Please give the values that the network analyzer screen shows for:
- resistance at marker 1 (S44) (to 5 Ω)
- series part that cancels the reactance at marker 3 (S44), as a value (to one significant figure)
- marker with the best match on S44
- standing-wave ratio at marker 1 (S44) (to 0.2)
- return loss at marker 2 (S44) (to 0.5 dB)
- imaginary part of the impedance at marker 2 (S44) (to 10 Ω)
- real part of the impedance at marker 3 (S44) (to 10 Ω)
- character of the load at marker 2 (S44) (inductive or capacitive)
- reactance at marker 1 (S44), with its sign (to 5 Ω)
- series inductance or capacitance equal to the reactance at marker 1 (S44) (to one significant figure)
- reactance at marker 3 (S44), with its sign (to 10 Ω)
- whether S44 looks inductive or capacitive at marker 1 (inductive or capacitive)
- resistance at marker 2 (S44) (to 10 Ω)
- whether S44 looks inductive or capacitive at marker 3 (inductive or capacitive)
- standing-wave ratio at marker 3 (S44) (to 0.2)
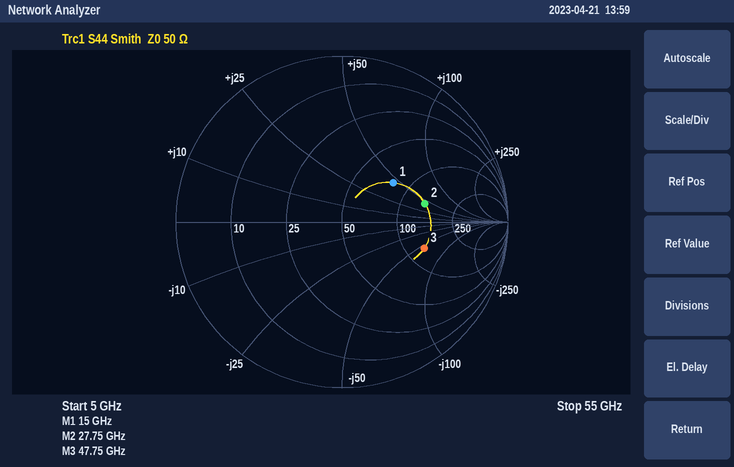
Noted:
80 Ω
200 pH
marker 1
2.2
6.0 dB
+40 Ω
130 Ω
inductive
+45 Ω
500 pH
-60 Ω
inductive
140 Ω
capacitive
3.2
